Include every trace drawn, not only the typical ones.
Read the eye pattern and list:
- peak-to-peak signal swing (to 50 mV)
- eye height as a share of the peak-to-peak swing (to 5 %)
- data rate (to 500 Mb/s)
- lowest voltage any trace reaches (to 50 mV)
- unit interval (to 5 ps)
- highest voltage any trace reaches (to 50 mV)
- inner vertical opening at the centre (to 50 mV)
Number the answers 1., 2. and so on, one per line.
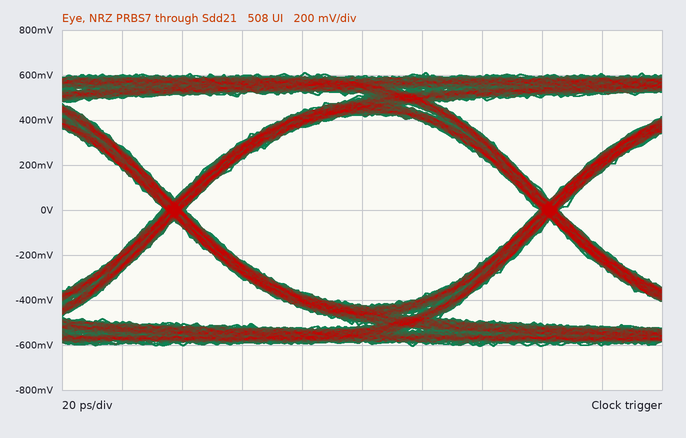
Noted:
1. 1.20 V
2. 70 %
3. 8.0 Gb/s
4. -600 mV
5. 125 ps
6. 600 mV
7. 850 mV
